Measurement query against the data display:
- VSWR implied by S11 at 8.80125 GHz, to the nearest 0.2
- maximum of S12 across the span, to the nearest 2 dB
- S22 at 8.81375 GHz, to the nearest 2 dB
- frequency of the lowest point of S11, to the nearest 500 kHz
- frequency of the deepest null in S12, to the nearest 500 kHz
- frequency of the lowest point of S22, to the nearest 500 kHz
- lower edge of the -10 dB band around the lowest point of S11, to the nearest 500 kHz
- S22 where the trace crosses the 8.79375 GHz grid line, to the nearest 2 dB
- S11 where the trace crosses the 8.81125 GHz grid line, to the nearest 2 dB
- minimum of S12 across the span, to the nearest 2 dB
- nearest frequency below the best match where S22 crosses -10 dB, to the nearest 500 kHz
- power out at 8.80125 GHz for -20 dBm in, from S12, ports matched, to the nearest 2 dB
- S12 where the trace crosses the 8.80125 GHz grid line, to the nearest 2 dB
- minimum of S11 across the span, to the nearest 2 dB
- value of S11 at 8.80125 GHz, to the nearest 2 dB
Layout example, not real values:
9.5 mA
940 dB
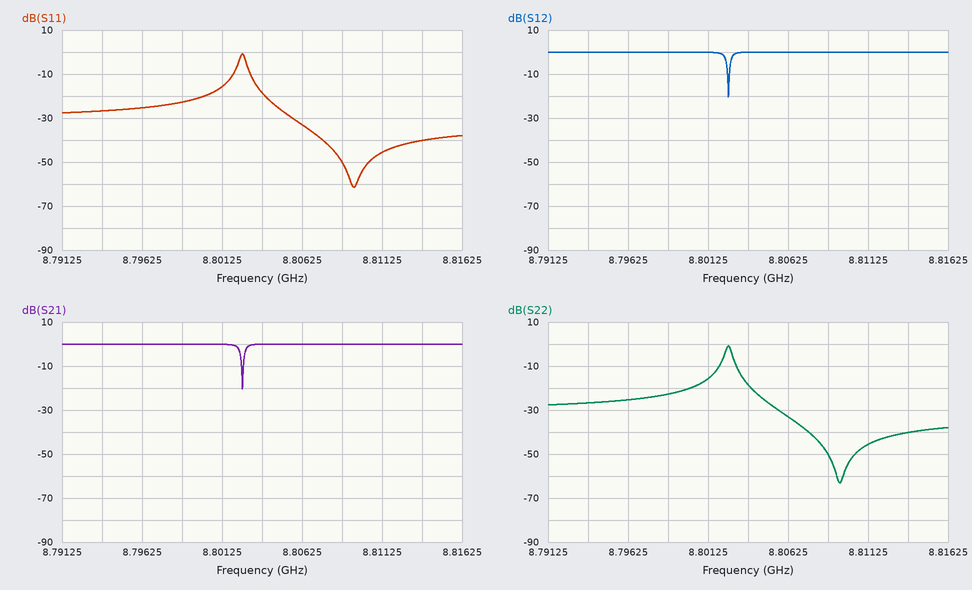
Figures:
1.4
0 dB
-40 dB
8.8095 GHz
8.8025 GHz
8.8095 GHz
8.8030 GHz
-26 dB
-46 dB
-20 dB
8.8030 GHz
-20 dBm
0 dB
-62 dB
-16 dB
